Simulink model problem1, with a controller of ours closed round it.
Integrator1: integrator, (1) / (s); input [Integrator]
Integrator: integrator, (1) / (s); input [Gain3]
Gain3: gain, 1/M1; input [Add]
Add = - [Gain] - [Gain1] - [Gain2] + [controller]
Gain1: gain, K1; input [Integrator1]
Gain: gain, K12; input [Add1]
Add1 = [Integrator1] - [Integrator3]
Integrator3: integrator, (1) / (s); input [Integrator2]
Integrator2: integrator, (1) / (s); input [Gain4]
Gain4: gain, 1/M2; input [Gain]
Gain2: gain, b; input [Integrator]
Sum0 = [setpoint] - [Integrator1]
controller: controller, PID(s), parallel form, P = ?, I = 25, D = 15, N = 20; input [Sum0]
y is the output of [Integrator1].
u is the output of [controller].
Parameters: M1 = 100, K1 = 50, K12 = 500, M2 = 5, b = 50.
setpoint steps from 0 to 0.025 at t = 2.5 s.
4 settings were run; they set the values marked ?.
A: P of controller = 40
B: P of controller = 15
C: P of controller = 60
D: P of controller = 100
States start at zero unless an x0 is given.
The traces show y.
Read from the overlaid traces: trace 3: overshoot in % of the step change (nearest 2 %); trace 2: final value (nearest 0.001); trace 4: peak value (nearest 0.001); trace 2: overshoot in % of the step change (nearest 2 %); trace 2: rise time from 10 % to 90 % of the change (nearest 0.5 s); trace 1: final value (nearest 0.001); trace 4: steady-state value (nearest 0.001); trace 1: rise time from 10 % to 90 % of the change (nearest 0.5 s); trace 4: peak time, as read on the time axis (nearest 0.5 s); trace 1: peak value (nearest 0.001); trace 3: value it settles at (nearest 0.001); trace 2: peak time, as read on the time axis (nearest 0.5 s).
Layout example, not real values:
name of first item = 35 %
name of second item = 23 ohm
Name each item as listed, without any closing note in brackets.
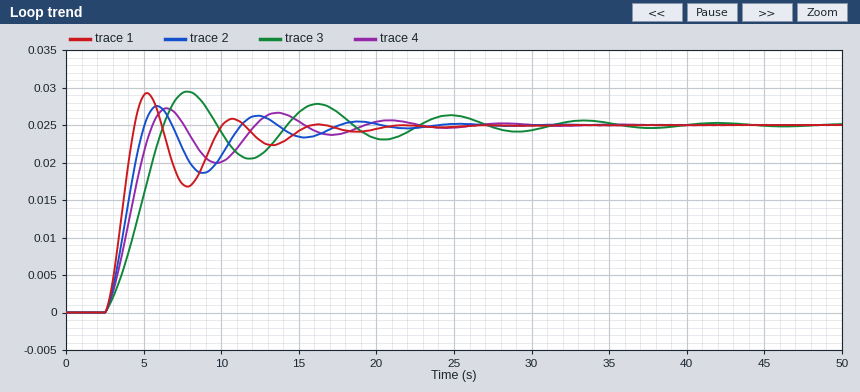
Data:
trace 3: overshoot in % of the step change = 18 %
trace 2: final value = 0.025
trace 4: peak value = 0.027
trace 2: overshoot in % of the step change = 10 %
trace 2: rise time from 10 % to 90 % of the change = 2.0 s
trace 1: final value = 0.025
trace 4: steady-state value = 0.025
trace 1: rise time from 10 % to 90 % of the change = 1.5 s
trace 4: peak time, as read on the time axis = 6.5 s
trace 1: peak value = 0.029
trace 3: value it settles at = 0.025
trace 2: peak time, as read on the time axis = 6.0 s
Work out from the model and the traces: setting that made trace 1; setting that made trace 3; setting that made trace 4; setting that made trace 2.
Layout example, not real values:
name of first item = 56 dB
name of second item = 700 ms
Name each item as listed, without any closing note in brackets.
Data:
setting that made trace 1 = D
setting that made trace 3 = B
setting that made trace 4 = A
setting that made trace 2 = C
